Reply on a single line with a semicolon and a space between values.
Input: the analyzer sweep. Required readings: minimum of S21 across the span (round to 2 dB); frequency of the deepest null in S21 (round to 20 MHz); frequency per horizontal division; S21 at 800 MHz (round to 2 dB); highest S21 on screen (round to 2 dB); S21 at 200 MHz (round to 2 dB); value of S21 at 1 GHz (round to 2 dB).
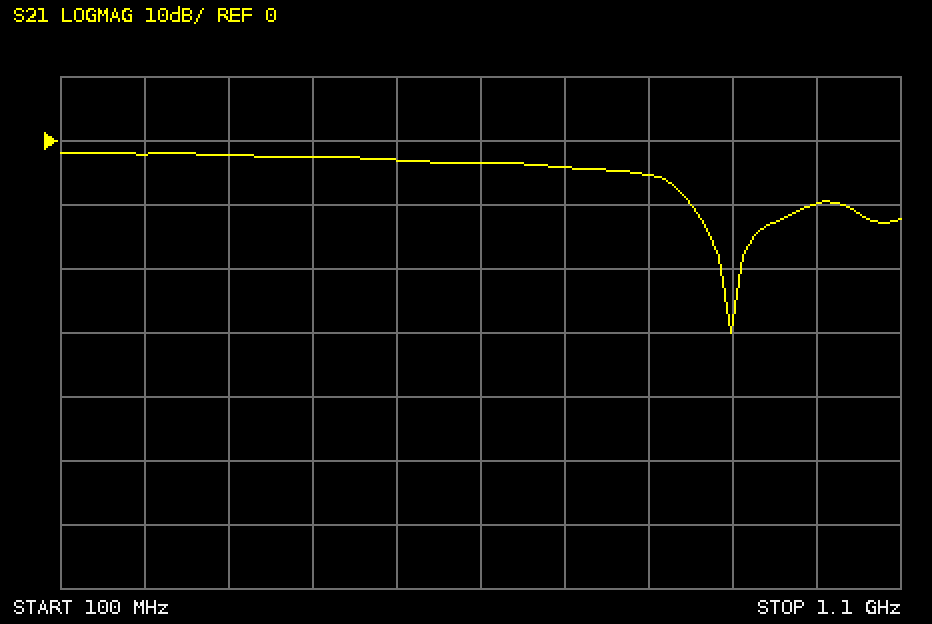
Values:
-30 dB; 900 MHz; 100 MHz; -6 dB; -2 dB; -2 dB; -10 dB
